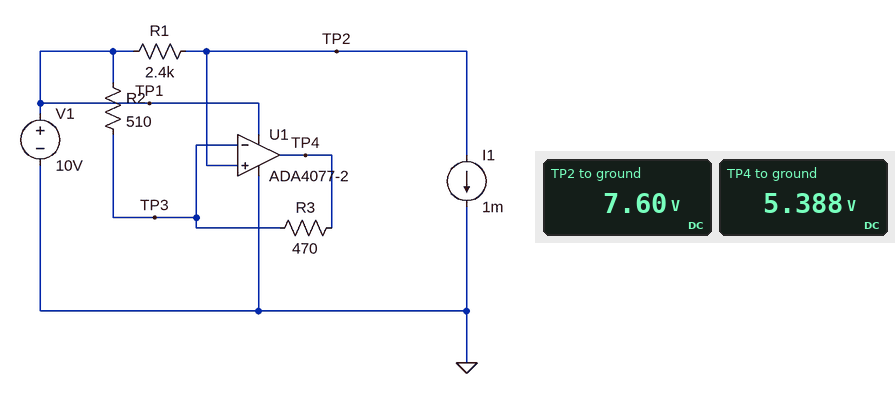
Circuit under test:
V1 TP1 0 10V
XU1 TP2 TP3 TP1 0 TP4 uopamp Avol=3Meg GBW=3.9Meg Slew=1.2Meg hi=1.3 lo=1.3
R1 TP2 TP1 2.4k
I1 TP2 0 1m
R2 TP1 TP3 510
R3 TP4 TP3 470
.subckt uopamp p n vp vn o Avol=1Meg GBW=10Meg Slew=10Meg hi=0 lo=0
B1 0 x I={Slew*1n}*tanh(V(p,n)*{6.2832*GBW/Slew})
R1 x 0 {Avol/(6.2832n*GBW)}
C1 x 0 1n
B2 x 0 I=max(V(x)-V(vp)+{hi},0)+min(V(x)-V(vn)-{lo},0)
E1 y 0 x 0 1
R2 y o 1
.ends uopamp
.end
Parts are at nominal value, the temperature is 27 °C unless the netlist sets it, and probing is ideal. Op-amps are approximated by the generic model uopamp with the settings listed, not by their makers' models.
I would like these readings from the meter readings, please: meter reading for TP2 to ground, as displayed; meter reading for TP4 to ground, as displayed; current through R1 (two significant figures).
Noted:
7.60 V
5.388 V
1.0 mA
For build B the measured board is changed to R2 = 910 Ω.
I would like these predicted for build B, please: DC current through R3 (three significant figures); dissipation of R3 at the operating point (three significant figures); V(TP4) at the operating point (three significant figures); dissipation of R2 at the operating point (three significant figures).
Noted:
2.64 mA
3.27 mW
6.36 V
6.33 mW
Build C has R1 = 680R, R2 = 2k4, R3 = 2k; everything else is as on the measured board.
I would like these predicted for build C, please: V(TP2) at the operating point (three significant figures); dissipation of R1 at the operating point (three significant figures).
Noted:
9.32 V
680 µW
